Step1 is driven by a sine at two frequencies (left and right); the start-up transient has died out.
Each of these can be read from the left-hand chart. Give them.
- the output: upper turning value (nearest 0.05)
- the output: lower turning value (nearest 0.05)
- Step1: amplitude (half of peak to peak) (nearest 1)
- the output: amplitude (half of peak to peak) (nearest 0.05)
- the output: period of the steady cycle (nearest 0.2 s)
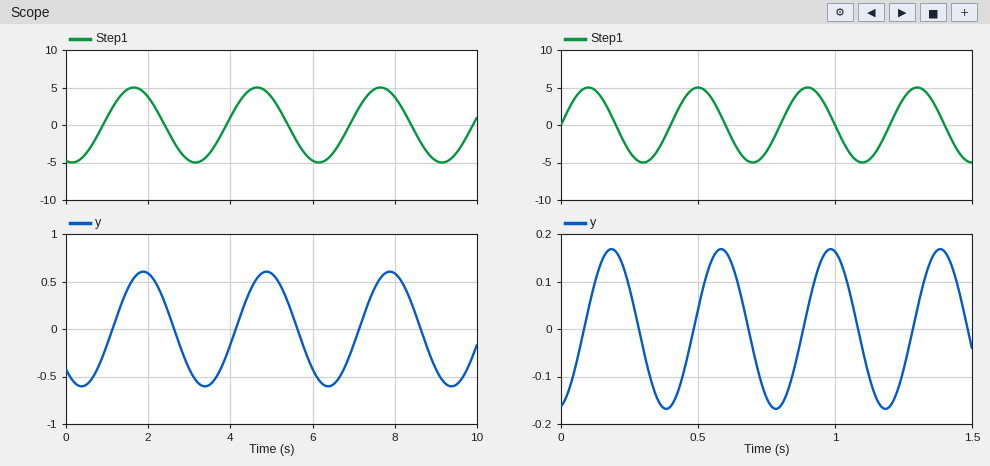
0.60
-0.60
5
0.60
3.0 s
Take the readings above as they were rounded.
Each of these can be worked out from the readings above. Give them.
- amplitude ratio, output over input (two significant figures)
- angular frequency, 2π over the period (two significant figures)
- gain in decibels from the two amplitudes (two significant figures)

0.12
2.1 rad/s
-18 dB
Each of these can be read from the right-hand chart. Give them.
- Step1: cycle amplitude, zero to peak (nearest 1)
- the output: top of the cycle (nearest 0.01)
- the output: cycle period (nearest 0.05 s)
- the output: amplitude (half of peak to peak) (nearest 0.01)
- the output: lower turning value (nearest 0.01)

5
0.17
0.40 s
0.17
-0.17
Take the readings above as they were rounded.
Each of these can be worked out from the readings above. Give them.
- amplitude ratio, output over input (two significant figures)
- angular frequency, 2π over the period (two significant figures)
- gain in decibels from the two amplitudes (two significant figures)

0.034
16 rad/s
-29 dB
